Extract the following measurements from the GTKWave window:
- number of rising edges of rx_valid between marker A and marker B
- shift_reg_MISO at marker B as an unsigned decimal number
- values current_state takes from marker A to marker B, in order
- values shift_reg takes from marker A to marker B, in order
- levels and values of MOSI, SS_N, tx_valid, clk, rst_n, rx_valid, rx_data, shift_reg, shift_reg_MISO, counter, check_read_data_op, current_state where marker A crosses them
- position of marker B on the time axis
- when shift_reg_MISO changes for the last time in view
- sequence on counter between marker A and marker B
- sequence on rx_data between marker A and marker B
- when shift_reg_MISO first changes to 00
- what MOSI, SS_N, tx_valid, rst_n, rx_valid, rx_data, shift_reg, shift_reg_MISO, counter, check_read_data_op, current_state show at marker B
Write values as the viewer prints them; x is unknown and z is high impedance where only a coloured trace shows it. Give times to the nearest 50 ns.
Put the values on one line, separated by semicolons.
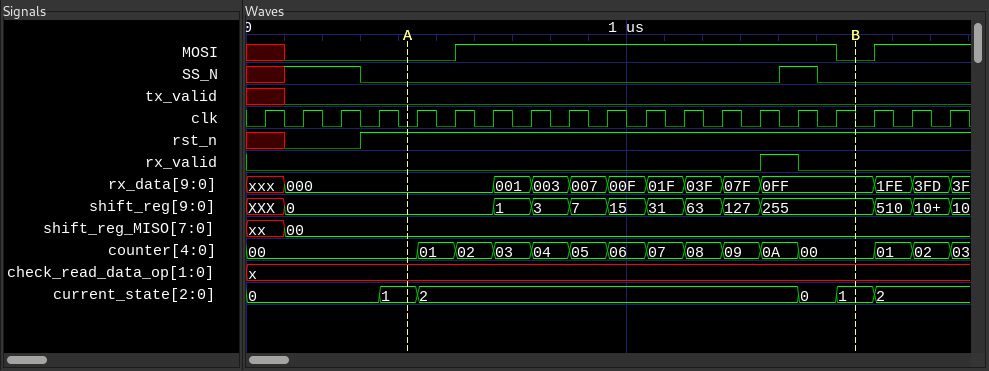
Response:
1; 0; 1, 2, 0, 1; 0, 1, 3, 7, 15, 31, 63, 127, 255; MOSI=0, SS_N=0, tx_valid=0, clk=0, rst_n=1, rx_valid=0, rx_data=000, shift_reg=0, shift_reg_MISO=00, counter=00, check_read_data_op=x, current_state=1; 1600 ns; 100 ns; 00, 01, 02, 03, 04, 05, 06, 07, 08, 09, 0A, 00; 000, 001, 003, 007, 00F, 01F, 03F, 07F, 0FF; 100 ns; MOSI=0, SS_N=0, tx_valid=0, rst_n=1, rx_valid=0, rx_data=0FF, shift_reg=255, shift_reg_MISO=00, counter=00, check_read_data_op=x, current_state=1
